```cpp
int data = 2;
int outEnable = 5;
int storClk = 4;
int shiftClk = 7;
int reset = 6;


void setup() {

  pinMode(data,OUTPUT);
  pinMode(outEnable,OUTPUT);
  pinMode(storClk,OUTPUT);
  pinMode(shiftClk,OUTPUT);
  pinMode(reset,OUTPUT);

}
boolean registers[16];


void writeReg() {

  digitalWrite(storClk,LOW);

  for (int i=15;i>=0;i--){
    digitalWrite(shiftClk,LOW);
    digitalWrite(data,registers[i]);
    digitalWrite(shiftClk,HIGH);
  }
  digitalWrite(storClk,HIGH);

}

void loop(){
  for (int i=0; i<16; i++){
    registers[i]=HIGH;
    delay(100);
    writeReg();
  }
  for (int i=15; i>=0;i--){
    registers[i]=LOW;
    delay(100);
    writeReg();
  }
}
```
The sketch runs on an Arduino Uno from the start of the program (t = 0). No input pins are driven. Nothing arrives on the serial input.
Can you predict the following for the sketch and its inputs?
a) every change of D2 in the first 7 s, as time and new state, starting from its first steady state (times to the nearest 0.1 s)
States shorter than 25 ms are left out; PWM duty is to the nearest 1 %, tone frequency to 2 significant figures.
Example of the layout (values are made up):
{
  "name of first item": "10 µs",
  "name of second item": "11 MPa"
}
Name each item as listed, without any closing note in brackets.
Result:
{
  "every change of D2 in the first 7 s, as time and new state, starting from its first steady state": "0 s low; 0.1 s high; 3.2 s low; 3.3 s high; 6.4 s low; 6.5 s high"
}
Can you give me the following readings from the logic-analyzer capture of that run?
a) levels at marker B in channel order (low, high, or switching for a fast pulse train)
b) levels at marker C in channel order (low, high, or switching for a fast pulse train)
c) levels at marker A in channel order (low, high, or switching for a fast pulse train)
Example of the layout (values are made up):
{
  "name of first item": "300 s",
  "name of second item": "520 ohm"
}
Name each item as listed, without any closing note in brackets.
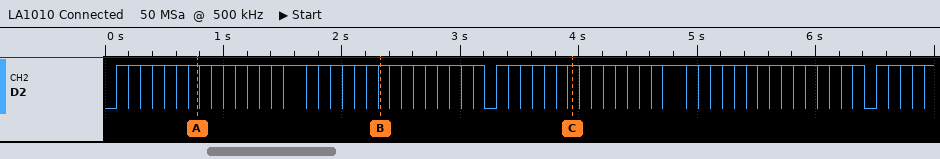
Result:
{
  "levels at marker B in channel order": "D2 high",
  "levels at marker C in channel order": "D2 high",
  "levels at marker A in channel order": "D2 high"
}
